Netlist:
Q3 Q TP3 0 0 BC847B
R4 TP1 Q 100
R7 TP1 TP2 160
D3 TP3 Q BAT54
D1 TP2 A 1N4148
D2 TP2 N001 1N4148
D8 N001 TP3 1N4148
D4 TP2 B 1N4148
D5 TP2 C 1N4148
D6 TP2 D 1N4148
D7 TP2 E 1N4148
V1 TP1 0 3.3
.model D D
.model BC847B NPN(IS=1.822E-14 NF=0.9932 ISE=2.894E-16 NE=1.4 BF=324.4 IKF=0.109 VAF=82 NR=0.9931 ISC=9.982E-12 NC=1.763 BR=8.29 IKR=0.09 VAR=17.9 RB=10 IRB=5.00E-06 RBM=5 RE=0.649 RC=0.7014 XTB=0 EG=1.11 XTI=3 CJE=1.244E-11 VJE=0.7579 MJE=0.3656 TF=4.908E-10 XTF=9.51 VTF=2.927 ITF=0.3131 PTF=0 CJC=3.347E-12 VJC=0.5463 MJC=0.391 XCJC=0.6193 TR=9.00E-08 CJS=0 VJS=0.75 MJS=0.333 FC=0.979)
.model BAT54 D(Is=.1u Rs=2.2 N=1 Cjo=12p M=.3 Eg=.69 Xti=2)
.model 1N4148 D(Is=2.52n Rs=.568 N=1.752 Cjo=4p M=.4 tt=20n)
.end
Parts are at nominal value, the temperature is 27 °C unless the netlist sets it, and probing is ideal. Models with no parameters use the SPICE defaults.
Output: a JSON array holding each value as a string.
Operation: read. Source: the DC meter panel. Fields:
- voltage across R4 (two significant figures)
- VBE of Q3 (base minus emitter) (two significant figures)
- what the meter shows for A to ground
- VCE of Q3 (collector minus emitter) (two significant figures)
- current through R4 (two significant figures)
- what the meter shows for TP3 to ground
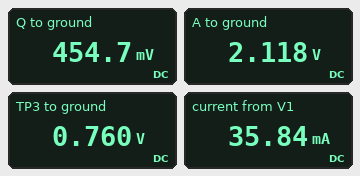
["2.8 V", "760 mV", "2.118 V", "450 mV", "28 mA", "0.760 V"]
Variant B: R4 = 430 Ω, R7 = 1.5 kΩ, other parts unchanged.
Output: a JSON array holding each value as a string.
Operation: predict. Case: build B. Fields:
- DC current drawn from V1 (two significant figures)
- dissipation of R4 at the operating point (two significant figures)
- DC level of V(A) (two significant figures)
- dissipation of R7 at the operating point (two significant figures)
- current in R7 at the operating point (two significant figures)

["7.6 mA", "19 mW", "1.9 V", "1.4 mW", "960 µA"]
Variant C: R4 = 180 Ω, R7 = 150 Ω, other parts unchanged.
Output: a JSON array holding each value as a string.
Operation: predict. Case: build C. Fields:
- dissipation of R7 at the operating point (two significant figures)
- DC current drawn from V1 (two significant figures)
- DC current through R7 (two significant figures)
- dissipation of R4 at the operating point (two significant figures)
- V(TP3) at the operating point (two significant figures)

["9.5 mW", "24 mA", "8.0 mA", "46 mW", "740 mV"]
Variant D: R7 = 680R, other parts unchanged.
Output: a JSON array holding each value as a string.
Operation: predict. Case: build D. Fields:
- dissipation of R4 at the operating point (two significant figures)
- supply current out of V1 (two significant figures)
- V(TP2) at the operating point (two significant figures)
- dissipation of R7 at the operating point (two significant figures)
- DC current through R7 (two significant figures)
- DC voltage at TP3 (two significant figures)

["79 mW", "30 mA", "2.0 V", "2.6 mW", "1.9 mA", "750 mV"]
